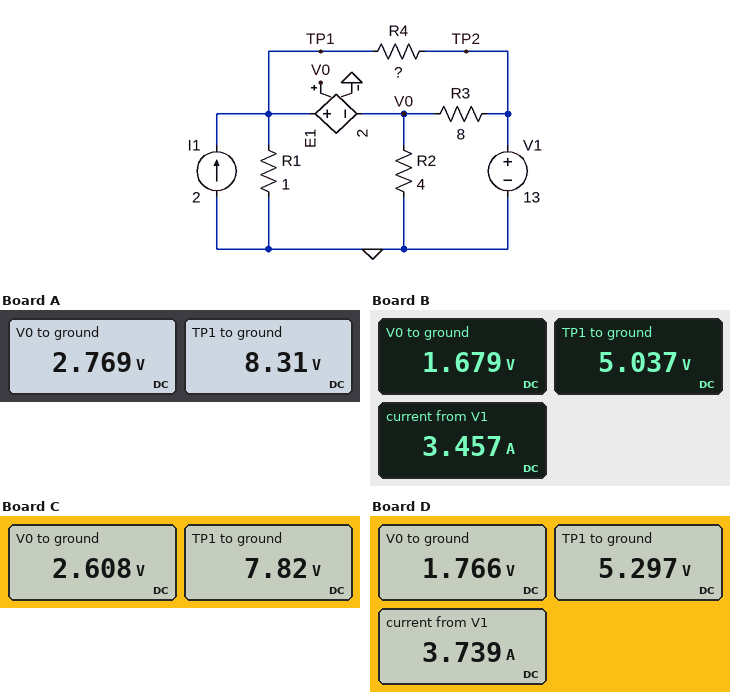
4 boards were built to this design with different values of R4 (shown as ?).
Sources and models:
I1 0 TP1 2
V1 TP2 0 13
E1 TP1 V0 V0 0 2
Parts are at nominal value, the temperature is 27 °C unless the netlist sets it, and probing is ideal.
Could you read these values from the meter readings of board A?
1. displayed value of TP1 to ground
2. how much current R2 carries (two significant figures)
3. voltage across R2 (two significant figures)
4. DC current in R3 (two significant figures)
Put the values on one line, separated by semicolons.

8.31 V; 690 mA; 2.8 V; 1.3 A
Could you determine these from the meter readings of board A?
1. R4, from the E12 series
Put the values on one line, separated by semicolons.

0.82 Ω
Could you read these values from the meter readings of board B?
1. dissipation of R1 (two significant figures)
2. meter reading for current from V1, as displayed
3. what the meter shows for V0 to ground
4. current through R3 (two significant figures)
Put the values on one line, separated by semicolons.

25 W; 3.457 A; 1.679 V; 1.4 A
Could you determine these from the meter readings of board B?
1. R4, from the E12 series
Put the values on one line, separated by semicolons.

3.9 Ω
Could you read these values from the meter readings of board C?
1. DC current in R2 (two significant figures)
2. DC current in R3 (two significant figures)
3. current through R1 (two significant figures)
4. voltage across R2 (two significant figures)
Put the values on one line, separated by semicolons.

650 mA; 1.3 A; 7.8 A; 2.6 V
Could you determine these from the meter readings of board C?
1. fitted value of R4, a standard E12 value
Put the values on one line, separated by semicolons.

1 Ω
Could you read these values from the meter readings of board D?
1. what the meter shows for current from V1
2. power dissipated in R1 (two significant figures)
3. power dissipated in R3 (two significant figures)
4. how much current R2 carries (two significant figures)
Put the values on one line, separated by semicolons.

3.739 A; 28 W; 16 W; 440 mA
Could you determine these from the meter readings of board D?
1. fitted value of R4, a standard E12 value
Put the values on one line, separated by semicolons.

3.3 Ω
